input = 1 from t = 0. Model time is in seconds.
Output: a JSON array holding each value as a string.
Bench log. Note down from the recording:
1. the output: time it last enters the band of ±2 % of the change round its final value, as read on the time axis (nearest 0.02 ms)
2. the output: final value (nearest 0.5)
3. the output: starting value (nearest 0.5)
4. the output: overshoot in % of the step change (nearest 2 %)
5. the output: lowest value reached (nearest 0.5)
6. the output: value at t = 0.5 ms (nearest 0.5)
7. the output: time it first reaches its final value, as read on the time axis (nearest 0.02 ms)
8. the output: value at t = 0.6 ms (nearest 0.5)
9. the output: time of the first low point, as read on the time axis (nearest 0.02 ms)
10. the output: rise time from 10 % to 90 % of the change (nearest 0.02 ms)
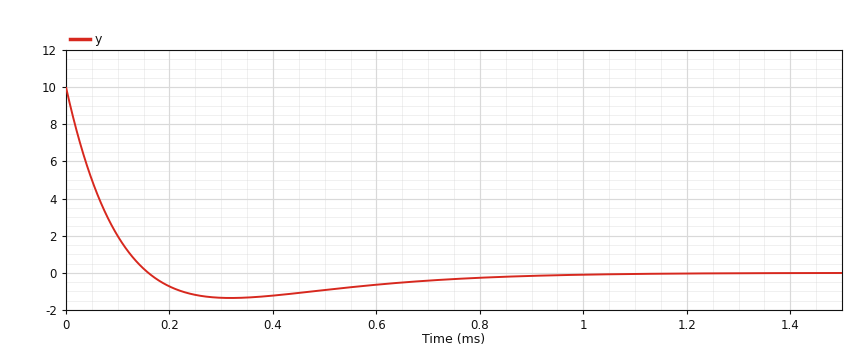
["0.86 ms", "0.0", "10.0", "14 %", "-1.5", "-1.0", "0.16 ms", "-0.5", "0.32 ms", "0.12 ms"]
